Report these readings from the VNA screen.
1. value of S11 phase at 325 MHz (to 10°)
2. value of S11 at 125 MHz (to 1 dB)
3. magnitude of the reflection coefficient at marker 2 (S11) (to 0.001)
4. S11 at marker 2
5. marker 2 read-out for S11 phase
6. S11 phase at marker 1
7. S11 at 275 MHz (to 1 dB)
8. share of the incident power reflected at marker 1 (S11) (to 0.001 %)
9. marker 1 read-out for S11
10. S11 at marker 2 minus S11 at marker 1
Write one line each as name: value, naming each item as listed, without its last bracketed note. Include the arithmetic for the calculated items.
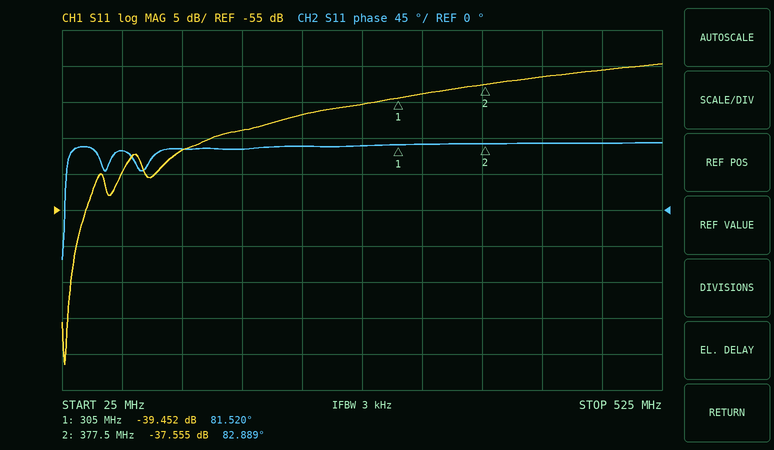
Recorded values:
value of S11 phase at 325 MHz: 80°
value of S11 at 125 MHz: -47 dB
magnitude of the reflection coefficient at marker 2 (S11): 10^(-37.555/20) ≈ 0.013
S11 at marker 2: -37.555 dB
marker 2 read-out for S11 phase: 82.889°
S11 phase at marker 1: 81.520°
S11 at 275 MHz: -40 dB
share of the incident power reflected at marker 1 (S11): 10^(-39.452/10) ≈ 0.011 %
marker 1 read-out for S11: -39.452 dB
S11 at marker 2 minus S11 at marker 1: -37.555 − (-39.452) = 1.897 dB
